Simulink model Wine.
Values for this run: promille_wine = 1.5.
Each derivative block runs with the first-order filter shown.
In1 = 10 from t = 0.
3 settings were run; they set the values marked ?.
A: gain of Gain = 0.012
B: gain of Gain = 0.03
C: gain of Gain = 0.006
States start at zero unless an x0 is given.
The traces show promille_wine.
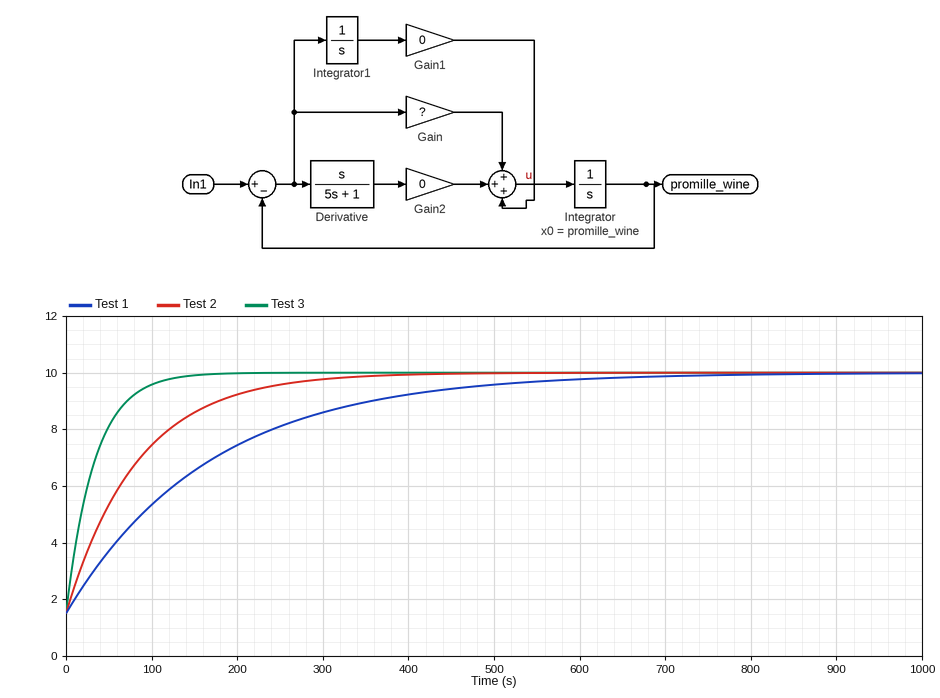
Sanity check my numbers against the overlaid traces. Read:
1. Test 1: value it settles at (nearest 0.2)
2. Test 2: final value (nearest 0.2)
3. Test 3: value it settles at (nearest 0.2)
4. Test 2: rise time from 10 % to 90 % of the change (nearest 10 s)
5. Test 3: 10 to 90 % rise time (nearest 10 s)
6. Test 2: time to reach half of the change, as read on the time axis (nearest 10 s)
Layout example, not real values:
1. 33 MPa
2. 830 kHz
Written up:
1. 10.0
2. 10.0
3. 10.0
4. 180 s
5. 70 s
6. 60 s
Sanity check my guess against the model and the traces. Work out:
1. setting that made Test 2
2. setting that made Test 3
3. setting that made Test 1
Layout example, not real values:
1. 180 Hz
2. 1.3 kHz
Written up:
1. A
2. B
3. C
